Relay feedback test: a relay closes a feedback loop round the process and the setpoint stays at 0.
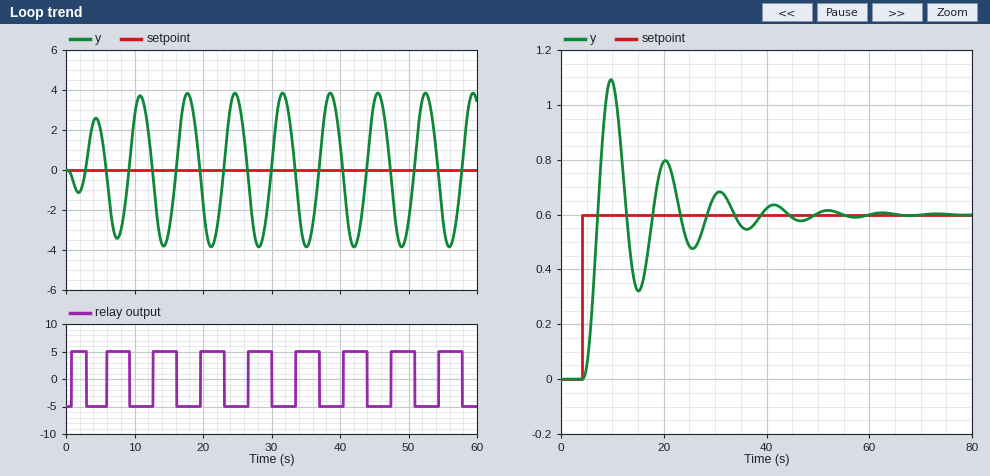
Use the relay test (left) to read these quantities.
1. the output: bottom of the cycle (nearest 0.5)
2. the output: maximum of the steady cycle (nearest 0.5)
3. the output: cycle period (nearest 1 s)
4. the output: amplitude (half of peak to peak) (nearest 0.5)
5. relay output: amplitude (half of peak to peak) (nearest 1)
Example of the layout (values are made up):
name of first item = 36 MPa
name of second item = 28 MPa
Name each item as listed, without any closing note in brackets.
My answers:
the output: bottom of the cycle = -4.0
the output: maximum of the steady cycle = 4.0
the output: cycle period = 7 s
the output: amplitude (half of peak to peak) = 4.0
relay output: amplitude (half of peak to peak) = 5
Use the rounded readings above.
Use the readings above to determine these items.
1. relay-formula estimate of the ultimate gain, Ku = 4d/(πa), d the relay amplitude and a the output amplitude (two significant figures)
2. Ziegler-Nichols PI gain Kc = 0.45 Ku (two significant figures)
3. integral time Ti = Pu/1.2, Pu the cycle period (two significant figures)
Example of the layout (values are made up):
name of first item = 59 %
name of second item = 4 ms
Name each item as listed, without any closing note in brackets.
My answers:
relay-formula estimate of the ultimate gain, Ku = 4d/(πa), d the relay amplitude and a the output amplitude = 1.6
Ziegler-Nichols PI gain Kc = 0.45 Ku = 0.72
integral time Ti = Pu/1.2, Pu the cycle period = 5.8 s
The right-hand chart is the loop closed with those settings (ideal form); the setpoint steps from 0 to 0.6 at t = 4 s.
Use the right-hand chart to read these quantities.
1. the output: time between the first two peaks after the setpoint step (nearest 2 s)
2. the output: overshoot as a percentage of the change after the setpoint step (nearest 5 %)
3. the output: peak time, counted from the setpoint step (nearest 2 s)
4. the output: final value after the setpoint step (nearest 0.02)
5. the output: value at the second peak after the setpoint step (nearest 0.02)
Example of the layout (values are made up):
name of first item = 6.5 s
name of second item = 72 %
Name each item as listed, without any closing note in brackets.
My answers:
the output: time between the first two peaks after the setpoint step = 10 s
the output: overshoot as a percentage of the change after the setpoint step = 80 %
the output: peak time, counted from the setpoint step = 6 s
the output: final value after the setpoint step = 0.60
the output: value at the second peak after the setpoint step = 0.80
